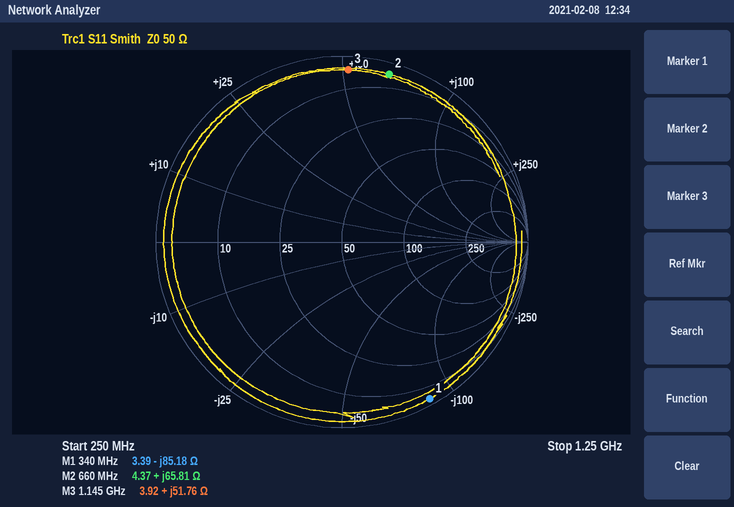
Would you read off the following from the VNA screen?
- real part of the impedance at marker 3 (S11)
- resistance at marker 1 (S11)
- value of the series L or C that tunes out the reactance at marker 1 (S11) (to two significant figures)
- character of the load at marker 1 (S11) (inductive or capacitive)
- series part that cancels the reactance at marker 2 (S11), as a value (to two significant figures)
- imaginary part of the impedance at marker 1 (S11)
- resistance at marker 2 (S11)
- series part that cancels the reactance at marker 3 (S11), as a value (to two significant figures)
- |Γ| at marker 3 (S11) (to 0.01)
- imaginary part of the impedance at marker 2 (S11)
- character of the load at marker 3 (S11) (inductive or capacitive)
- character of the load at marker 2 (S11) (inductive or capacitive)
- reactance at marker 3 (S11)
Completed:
3.92 Ω
3.39 Ω
40 nH
capacitive
3.7 pF
-85.18 Ω
4.37 Ω
2.7 pF
0.93
+65.81 Ω
inductive
inductive
+51.76 Ω
